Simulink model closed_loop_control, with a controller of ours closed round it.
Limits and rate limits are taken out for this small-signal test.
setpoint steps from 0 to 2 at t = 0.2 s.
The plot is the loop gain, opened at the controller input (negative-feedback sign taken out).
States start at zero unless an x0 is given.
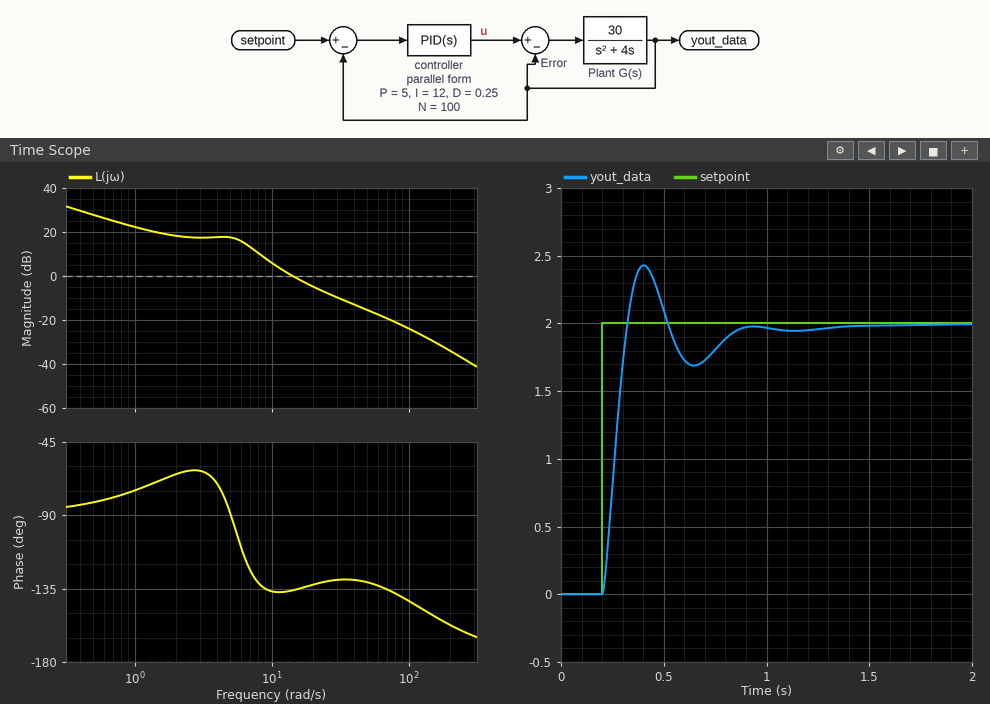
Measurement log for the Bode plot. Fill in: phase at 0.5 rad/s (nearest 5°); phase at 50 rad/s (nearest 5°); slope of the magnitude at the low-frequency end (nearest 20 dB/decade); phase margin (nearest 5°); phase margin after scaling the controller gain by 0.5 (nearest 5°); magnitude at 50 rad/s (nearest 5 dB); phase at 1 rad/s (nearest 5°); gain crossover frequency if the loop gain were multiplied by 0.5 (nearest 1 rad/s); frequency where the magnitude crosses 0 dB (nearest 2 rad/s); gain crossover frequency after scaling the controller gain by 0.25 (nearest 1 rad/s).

-80°
-130°
-20 dB/decade
45°
45°
-15 dB
-75°
10 rad/s
14 rad/s
7 rad/s
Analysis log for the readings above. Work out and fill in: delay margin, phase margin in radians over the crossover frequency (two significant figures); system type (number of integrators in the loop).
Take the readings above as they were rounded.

0.056 s
1
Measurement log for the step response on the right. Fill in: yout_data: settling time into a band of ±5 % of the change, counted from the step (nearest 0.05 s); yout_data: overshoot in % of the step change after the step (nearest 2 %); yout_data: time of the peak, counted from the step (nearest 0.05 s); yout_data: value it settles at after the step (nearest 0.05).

0.60 s
22 %
0.20 s
2.00
